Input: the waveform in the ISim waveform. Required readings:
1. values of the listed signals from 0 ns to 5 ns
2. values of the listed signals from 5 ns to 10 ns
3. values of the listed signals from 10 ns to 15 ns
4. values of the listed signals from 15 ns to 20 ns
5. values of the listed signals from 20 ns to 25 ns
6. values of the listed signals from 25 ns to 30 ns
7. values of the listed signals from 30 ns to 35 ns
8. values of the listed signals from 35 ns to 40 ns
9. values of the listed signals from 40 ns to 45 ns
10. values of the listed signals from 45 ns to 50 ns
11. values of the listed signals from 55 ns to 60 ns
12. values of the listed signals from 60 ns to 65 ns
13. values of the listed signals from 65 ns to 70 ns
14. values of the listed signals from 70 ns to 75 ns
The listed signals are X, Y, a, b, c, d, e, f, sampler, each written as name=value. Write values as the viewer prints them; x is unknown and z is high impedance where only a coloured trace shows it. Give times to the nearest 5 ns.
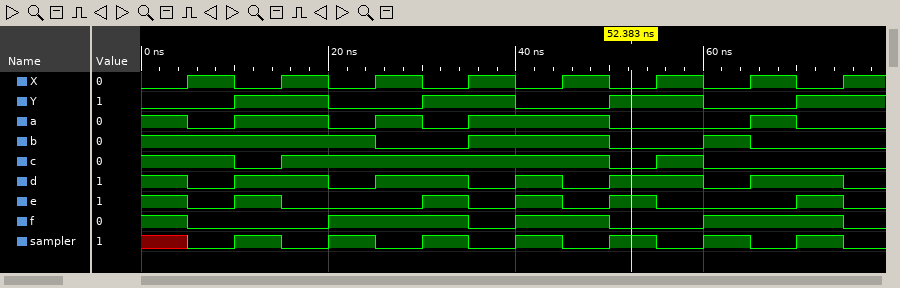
X=0, Y=0, a=1, b=1, c=1, d=1, e=1, f=1, sampler=x
X=1, Y=0, a=0, b=1, c=1, d=0, e=0, f=0, sampler=0
X=0, Y=1, a=1, b=1, c=0, d=1, e=1, f=0, sampler=1
X=1, Y=1, a=1, b=1, c=1, d=1, e=0, f=0, sampler=0
X=0, Y=0, a=0, b=1, c=1, d=0, e=0, f=1, sampler=1
X=1, Y=0, a=1, b=0, c=1, d=1, e=0, f=1, sampler=0
X=0, Y=1, a=0, b=0, c=1, d=1, e=1, f=1, sampler=1
X=1, Y=1, a=1, b=1, c=1, d=0, e=0, f=0, sampler=0
X=0, Y=0, a=1, b=1, c=1, d=1, e=1, f=1, sampler=1
X=1, Y=0, a=1, b=1, c=1, d=0, e=0, f=1, sampler=0
X=1, Y=1, a=0, b=0, c=1, d=1, e=0, f=0, sampler=0
X=0, Y=0, a=0, b=1, c=0, d=0, e=0, f=1, sampler=1
X=1, Y=0, a=1, b=0, c=0, d=1, e=0, f=1, sampler=0
X=0, Y=1, a=0, b=0, c=0, d=1, e=1, f=1, sampler=1
